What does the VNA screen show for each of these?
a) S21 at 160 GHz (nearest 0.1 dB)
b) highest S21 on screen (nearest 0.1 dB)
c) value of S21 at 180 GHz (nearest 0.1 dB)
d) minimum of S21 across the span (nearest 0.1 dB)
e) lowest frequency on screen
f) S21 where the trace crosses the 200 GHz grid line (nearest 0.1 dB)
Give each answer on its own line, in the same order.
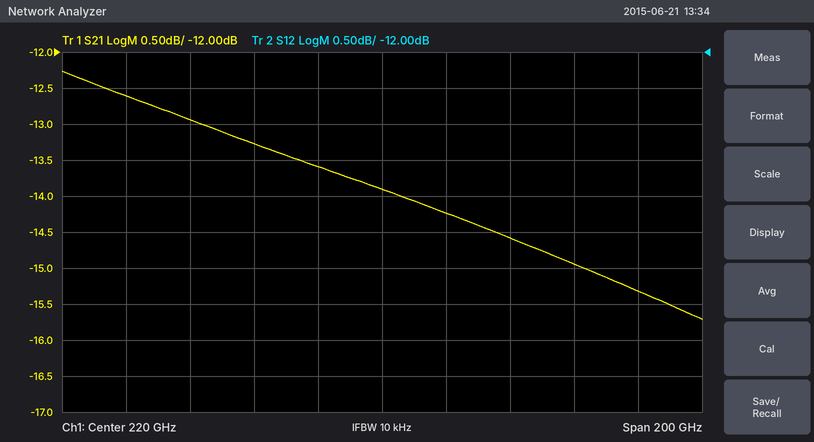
-12.9 dB
-12.3 dB
-13.3 dB
-15.7 dB
120 GHz
-13.6 dB
